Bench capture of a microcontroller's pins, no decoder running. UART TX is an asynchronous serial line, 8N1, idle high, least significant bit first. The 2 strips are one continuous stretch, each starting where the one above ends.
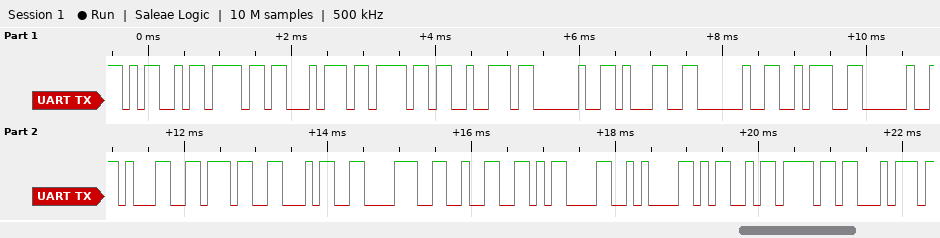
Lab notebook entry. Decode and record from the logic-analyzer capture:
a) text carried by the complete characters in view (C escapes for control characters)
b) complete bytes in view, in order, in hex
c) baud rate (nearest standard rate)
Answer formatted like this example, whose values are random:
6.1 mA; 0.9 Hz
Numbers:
"Motor 1 : 17482\r\nMot"; 4D 6F 74 6F 72 20 31 20 3A 20 31 37 34 38 32 0D 0A 4D 6F 74; 9600 baud
